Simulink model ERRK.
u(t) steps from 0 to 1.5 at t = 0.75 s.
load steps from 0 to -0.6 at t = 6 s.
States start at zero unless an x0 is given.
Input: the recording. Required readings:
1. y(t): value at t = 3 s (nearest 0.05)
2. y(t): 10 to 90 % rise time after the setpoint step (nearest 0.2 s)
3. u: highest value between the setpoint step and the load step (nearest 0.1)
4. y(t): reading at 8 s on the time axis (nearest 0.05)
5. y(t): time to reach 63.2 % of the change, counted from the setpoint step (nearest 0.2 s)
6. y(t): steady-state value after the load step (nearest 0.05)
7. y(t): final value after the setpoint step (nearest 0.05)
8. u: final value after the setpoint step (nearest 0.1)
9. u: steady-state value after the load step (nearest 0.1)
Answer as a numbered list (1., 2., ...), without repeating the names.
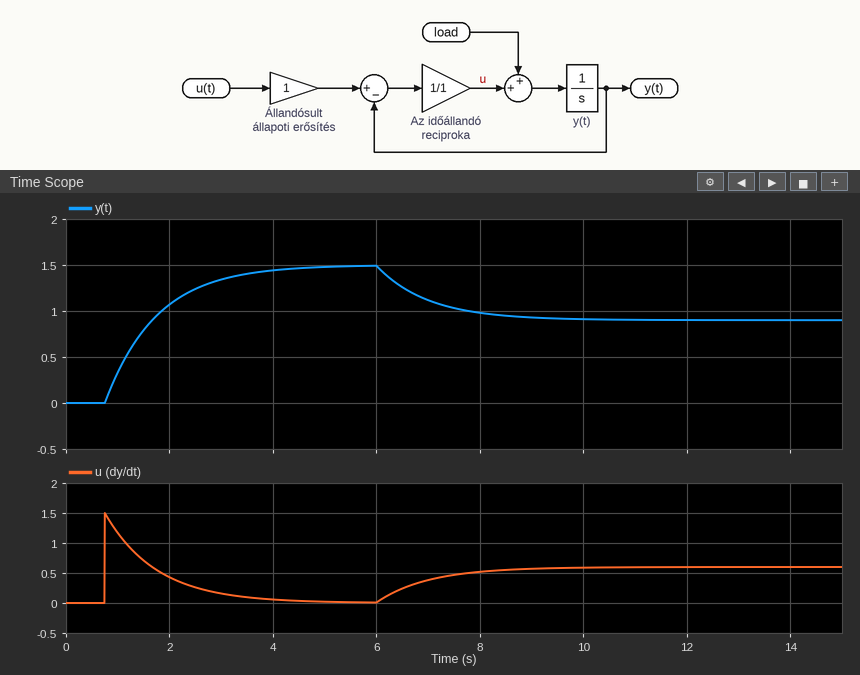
1. 1.35
2. 2.2 s
3. 1.5
4. 1.00
5. 1.0 s
6. 0.90
7. 1.50
8. 0.0
9. 0.6
